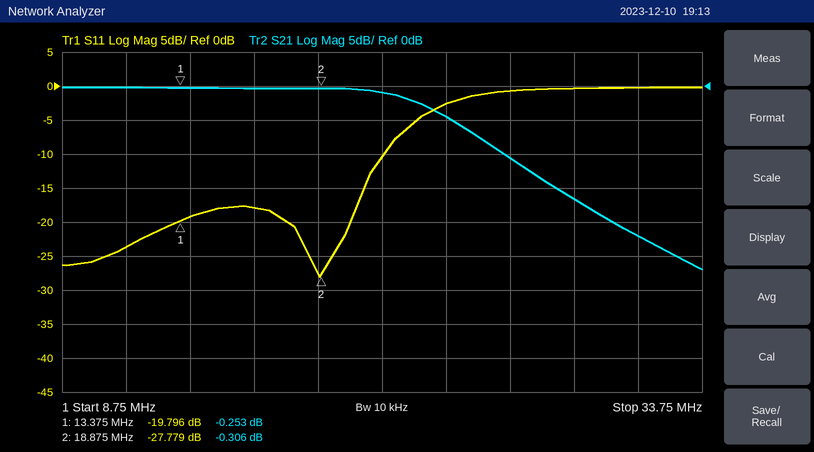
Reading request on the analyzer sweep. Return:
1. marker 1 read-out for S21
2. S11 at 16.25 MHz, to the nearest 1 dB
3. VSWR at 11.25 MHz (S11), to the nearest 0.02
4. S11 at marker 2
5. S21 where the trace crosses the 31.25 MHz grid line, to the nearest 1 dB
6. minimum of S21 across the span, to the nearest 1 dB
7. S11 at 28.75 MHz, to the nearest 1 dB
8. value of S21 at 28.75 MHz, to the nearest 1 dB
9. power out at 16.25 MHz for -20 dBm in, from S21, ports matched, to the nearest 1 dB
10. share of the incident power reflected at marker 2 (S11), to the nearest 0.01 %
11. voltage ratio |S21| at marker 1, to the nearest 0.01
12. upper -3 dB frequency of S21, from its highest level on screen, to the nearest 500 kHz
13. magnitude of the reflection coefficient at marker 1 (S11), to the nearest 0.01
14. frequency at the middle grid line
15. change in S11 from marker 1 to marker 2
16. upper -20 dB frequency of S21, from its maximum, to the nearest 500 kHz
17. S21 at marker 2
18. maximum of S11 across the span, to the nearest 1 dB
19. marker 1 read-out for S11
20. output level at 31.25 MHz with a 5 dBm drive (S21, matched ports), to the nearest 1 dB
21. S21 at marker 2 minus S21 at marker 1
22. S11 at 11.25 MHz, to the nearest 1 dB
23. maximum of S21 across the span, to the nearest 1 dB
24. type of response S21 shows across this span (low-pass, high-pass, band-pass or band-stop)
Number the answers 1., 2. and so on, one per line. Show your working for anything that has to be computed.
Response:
1. -0.253 dB
2. -18 dB
3. |Γ| = 10^(-24/20) = 0.0631; VSWR = (1 + 0.0631)/(1 − 0.0631) ≈ 1.13, so 1.14 to the nearest 0.02
4. -27.779 dB
5. -22 dB
6. -27 dB
7. 0 dB
8. -17 dB
9. -20 dBm + (0 dB) = -20 dBm
10. 10^(-27.779/10) ≈ 0.17 %
11. 10^(-0.253/20) ≈ 0.97
12. 23.0 MHz
13. 10^(-19.796/20) ≈ 0.10
14. 21.25 MHz
15. -27.779 − (-19.796) = -7.983 dB
16. 30.5 MHz
17. -0.306 dB
18. 0 dB
19. -19.796 dB
20. 5 dBm + (-22 dB) = -17 dBm
21. -0.306 − (-0.253) = -0.053 dB
22. -24 dB
23. 0 dB
24. low-pass
